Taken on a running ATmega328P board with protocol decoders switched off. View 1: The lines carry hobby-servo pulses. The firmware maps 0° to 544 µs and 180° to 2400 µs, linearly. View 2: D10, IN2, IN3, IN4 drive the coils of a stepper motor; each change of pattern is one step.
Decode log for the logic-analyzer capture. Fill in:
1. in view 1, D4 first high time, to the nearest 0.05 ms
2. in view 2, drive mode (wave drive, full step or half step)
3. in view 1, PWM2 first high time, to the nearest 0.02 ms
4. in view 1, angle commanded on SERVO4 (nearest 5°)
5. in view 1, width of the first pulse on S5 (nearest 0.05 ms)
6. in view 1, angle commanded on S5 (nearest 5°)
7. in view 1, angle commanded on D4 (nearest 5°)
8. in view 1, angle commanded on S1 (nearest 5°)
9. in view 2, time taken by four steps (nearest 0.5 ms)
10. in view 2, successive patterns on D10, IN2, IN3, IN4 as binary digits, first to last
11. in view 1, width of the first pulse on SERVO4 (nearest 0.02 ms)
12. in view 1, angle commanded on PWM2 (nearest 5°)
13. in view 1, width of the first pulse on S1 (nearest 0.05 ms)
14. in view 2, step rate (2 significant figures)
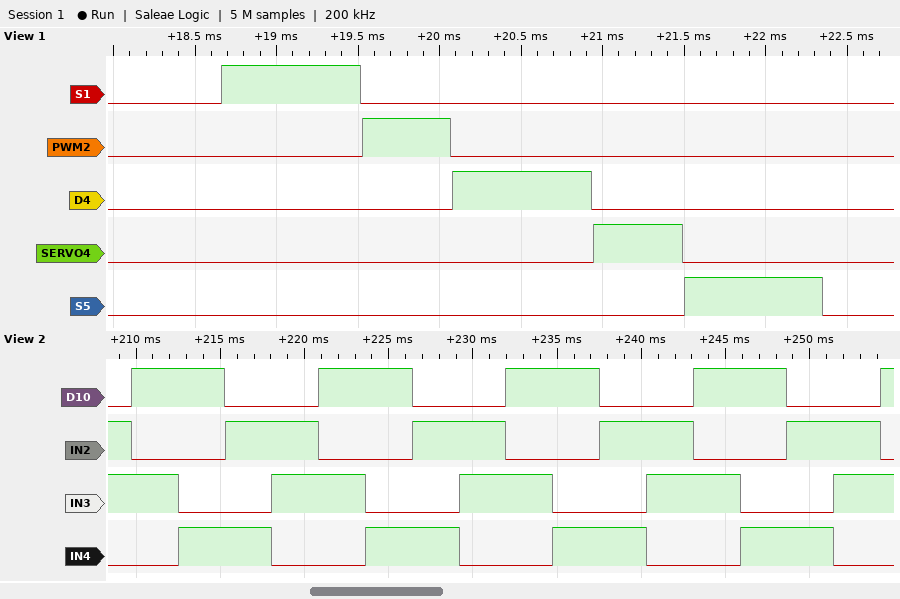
0.85 ms
full step
0.54 ms
0°
0.85 ms
30°
30°
30°
11.0 ms
0110 1010 1001 0101 0110 1010 1001 0101 0110 1010 1001 0101 0110 1010 1001 0101 0110 1010
0.54 ms
0°
0.85 ms
360 steps/s
